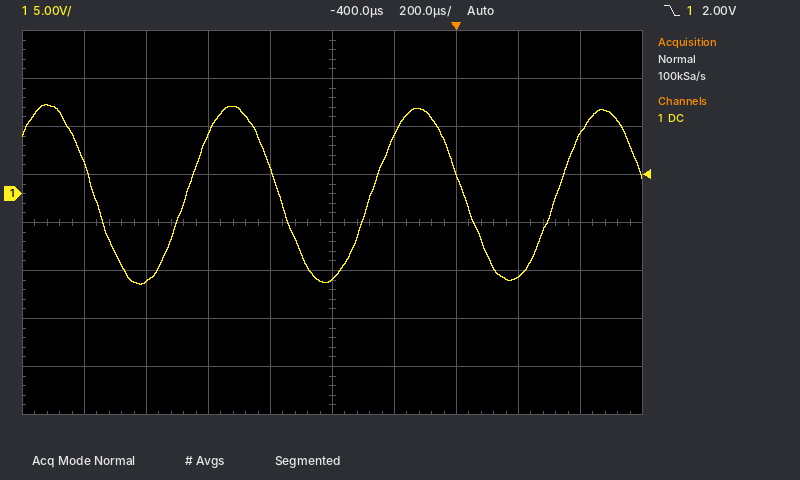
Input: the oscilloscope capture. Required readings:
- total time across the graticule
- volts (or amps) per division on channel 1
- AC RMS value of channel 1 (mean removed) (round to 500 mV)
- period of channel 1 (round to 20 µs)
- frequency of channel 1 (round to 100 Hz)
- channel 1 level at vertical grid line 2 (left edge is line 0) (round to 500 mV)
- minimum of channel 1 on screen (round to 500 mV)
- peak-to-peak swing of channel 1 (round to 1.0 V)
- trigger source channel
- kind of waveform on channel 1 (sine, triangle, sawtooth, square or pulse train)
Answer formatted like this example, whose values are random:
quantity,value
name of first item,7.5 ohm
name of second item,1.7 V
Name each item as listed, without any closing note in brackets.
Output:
quantity,value
total time across the graticule,2 ms
volts (or amps) per division on channel 1,5 V
AC RMS value of channel 1 (mean removed),6.5 V
period of channel 1,600 µs
frequency of channel 1,1.7 kHz
channel 1 level at vertical grid line 2 (left edge is line 0),-9.0 V
minimum of channel 1 on screen,-9.5 V
peak-to-peak swing of channel 1,19.0 V
trigger source channel,channel 1
kind of waveform on channel 1,sine
